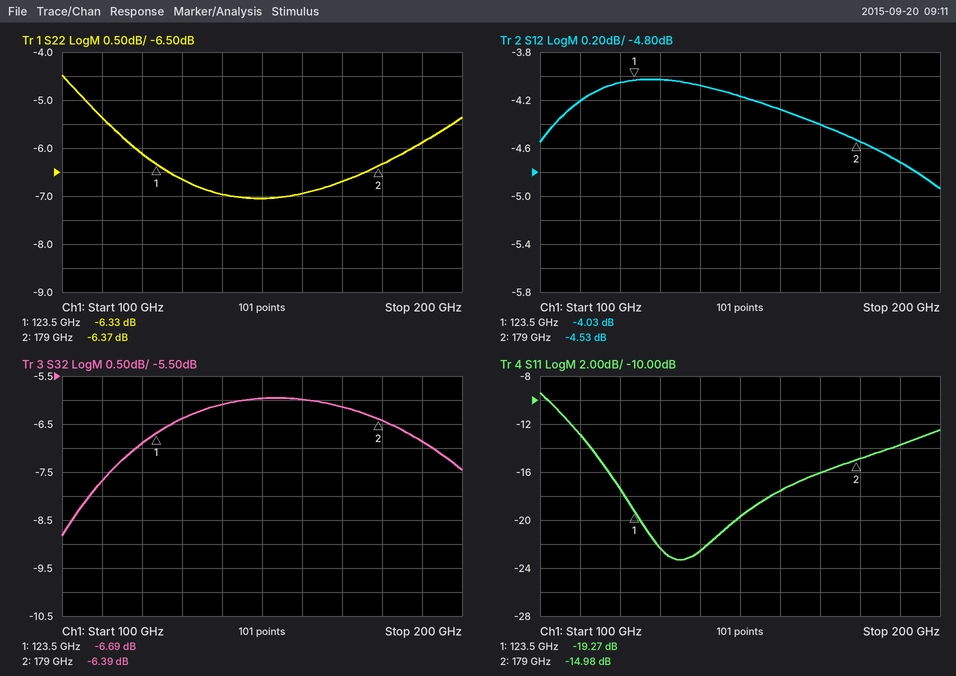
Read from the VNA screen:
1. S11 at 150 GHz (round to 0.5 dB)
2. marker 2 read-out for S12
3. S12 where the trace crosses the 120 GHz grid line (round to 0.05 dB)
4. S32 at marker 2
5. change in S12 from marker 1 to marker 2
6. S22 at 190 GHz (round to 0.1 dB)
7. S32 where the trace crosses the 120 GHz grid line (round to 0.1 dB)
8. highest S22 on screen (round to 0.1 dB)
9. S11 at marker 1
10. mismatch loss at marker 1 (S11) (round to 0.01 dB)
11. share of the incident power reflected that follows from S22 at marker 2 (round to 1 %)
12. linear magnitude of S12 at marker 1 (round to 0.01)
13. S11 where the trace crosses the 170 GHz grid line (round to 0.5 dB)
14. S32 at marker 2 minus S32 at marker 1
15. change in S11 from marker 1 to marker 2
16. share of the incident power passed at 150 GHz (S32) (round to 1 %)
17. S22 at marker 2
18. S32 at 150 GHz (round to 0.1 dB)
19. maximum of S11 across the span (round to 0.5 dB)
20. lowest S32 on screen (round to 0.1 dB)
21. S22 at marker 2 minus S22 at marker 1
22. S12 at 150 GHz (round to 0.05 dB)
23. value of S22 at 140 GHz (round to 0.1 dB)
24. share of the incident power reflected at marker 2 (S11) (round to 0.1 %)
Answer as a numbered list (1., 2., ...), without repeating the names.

1. -19.5 dB
2. -4.53 dB
3. -4.05 dB
4. -6.39 dB
5. -0.50 dB
6. -5.9 dB
7. -6.9 dB
8. -4.5 dB
9. -19.27 dB
10. 0.05 dB
11. 23 %
12. 0.63
13. -16.0 dB
14. 0.30 dB
15. 4.29 dB
16. 25 %
17. -6.37 dB
18. -6.0 dB
19. -9.5 dB
20. -8.8 dB
21. -0.04 dB
22. -4.15 dB
23. -7.0 dB
24. 3.2 %
